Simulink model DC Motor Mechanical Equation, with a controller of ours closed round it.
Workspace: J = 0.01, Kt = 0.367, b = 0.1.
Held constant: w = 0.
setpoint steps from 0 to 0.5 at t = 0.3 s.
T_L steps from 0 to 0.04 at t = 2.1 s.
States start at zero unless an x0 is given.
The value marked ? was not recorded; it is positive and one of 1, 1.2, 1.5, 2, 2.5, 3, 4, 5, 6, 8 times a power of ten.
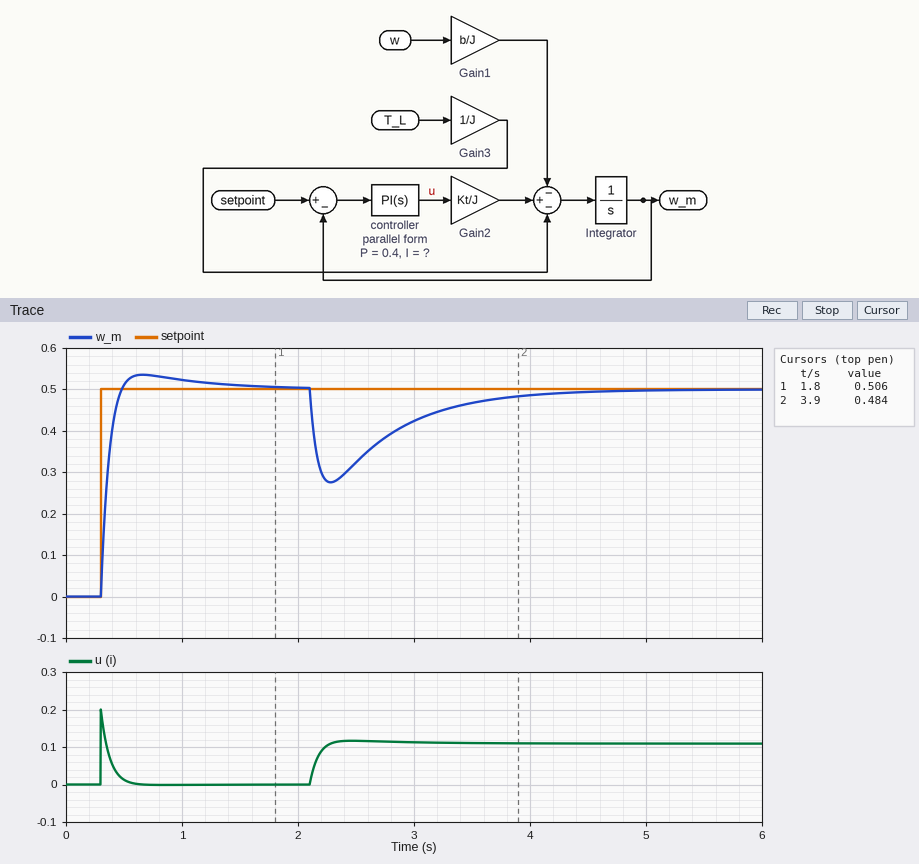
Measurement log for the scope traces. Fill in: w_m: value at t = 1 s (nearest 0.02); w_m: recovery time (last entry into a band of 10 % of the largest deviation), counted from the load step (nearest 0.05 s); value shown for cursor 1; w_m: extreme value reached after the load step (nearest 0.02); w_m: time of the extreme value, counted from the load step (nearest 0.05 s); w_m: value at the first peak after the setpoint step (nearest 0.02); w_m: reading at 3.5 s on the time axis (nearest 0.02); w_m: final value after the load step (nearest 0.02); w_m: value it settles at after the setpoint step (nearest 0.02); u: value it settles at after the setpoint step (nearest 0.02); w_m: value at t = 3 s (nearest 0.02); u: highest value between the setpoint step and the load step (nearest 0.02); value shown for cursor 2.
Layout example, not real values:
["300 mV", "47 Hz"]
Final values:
["0.52", "1.60 s", "0.506", "0.28", "0.20 s", "0.54", "0.46", "0.50", "0.50", "0.00", "0.42", "0.20", "0.484"]
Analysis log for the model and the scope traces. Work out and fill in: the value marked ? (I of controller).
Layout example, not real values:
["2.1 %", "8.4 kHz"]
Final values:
["0.6"]
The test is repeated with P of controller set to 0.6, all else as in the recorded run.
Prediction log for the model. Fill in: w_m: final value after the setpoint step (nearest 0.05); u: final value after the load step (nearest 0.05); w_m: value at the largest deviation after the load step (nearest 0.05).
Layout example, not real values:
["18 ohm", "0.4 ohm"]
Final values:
["0.50", "0.10", "0.35"]
